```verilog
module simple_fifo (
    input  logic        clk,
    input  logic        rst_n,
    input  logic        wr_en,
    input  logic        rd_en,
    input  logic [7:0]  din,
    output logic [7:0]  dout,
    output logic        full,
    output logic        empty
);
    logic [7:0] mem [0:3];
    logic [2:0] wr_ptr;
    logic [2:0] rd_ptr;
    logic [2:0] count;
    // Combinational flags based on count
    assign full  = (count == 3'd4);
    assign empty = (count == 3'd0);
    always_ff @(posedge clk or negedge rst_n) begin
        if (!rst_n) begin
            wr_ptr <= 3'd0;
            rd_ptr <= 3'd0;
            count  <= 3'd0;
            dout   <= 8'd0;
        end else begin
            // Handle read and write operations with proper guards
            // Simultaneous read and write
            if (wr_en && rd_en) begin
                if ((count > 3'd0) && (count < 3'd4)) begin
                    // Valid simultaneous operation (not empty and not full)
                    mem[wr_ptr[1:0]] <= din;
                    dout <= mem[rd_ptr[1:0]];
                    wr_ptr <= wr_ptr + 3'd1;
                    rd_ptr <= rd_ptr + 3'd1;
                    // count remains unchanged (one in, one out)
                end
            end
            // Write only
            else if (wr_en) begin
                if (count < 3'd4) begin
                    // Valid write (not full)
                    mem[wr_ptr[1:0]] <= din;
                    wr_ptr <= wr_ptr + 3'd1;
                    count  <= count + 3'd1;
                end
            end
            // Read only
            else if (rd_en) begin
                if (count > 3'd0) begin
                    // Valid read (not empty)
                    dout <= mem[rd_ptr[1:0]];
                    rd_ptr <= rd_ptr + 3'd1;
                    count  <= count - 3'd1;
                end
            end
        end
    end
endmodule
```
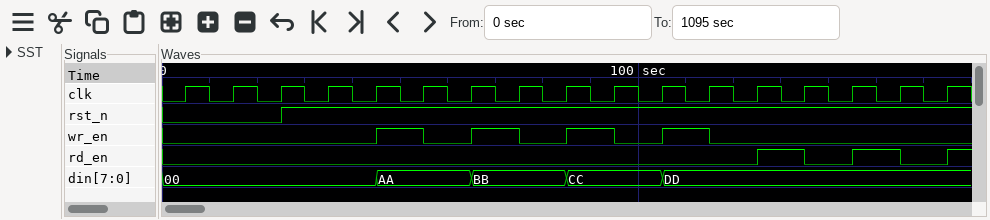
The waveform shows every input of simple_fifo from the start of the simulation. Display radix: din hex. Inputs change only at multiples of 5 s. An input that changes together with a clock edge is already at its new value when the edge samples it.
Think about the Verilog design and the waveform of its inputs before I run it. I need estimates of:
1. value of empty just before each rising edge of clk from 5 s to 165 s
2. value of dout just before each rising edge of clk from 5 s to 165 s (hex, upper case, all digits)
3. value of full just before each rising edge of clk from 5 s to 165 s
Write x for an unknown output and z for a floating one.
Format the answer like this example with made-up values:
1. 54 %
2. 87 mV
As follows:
1. 1 1 1 1 1 0 0 0 0 0 0 0 0 0 0 0 0
2. 00, 00, 00, 00, 00, 00, 00, 00, 00, 00, 00, 00, 00, AA, AA, BB, BB
3. 0 0 0 0 0 0 0 0 0 0 0 1 1 0 0 0 0
